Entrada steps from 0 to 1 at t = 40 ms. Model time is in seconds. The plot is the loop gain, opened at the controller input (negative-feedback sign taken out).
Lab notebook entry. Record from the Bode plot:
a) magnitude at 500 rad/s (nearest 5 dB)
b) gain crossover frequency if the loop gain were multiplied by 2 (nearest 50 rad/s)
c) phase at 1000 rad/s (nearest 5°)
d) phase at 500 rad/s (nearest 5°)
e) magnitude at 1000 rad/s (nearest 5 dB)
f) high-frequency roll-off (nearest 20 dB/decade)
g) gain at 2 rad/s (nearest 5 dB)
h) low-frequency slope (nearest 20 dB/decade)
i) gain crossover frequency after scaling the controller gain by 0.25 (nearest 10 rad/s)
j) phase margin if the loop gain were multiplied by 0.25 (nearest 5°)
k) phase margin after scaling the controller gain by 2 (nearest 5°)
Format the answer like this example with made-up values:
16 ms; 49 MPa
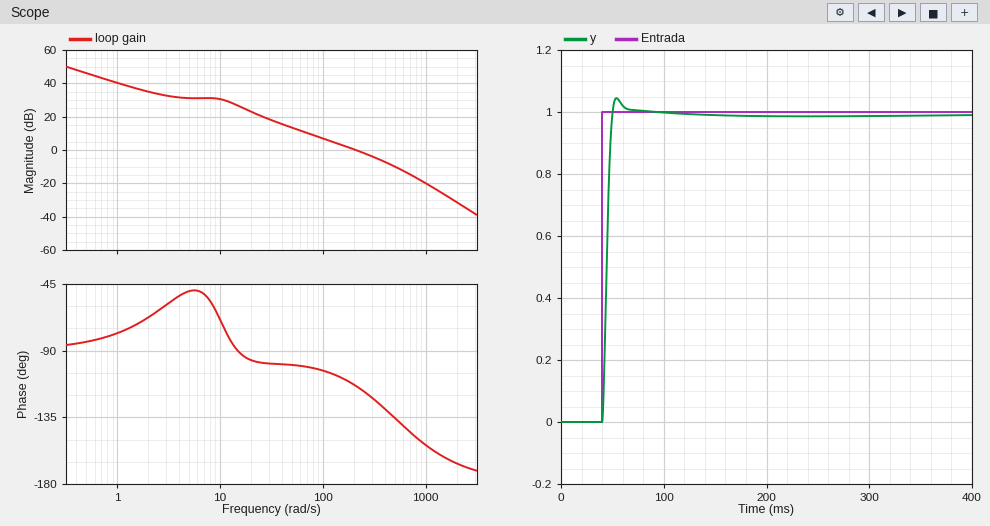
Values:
-10 dB; 350 rad/s; -155°; -135°; -20 dB; -40 dB/decade; 35 dB; -20 dB/decade; 60 rad/s; 80°; 55°
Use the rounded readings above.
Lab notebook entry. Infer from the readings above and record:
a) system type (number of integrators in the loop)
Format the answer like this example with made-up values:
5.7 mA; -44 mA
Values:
1
